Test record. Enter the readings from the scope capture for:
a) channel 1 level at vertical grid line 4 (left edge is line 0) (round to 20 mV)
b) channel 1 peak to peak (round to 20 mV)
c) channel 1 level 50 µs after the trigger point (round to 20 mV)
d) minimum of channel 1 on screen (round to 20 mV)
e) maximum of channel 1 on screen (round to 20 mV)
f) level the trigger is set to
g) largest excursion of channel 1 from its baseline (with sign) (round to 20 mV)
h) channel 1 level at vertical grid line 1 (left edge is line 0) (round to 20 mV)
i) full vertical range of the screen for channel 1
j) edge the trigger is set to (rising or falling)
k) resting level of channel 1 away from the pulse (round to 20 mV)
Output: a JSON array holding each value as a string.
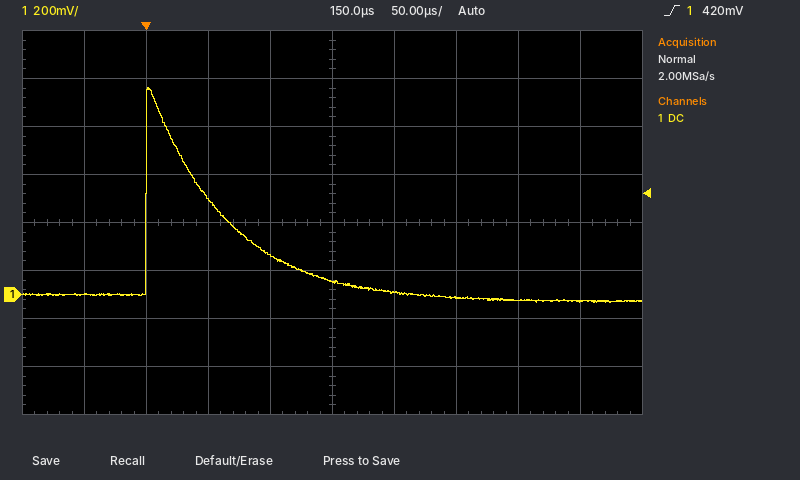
["160 mV", "900 mV", "400 mV", "-40 mV", "860 mV", "420 mV", "+860 mV", "0 mV", "1.6 V", "rising", "0 mV"]
